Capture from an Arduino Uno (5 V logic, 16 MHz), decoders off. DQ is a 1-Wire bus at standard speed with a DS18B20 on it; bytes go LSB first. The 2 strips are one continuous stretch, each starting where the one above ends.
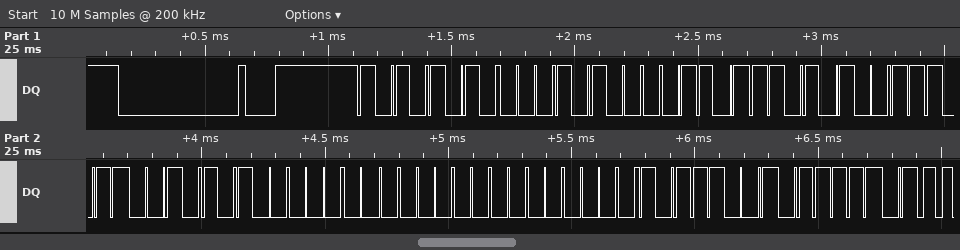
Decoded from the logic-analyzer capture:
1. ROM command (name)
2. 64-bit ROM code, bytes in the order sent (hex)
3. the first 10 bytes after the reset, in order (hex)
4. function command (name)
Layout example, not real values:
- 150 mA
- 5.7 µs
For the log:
- Match ROM
- 28 EC CA 4D 05 00 00 9D
- 55 28 EC CA 4D 05 00 00 9D BE
- Read Scratchpad
